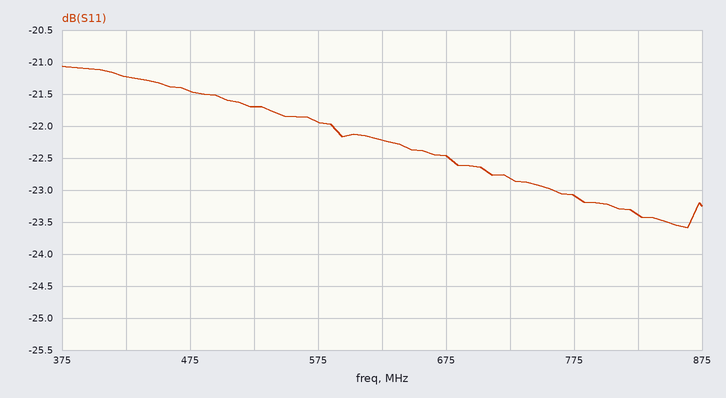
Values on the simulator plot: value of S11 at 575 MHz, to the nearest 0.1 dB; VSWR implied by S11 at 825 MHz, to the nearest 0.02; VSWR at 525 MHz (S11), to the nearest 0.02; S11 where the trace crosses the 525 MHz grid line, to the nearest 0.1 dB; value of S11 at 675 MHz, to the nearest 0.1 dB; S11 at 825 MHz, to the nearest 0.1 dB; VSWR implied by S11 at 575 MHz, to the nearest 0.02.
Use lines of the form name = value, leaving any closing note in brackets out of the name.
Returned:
value of S11 at 575 MHz, to the nearest 0.1 dB = -21.9 dB
VSWR implied by S11 at 825 MHz, to the nearest 0.02 = 1.14
VSWR at 525 MHz (S11), to the nearest 0.02 = 1.18
S11 where the trace crosses the 525 MHz grid line, to the nearest 0.1 dB = -21.7 dB
value of S11 at 675 MHz, to the nearest 0.1 dB = -22.5 dB
S11 at 825 MHz, to the nearest 0.1 dB = -23.4 dB
VSWR implied by S11 at 575 MHz, to the nearest 0.02 = 1.18
